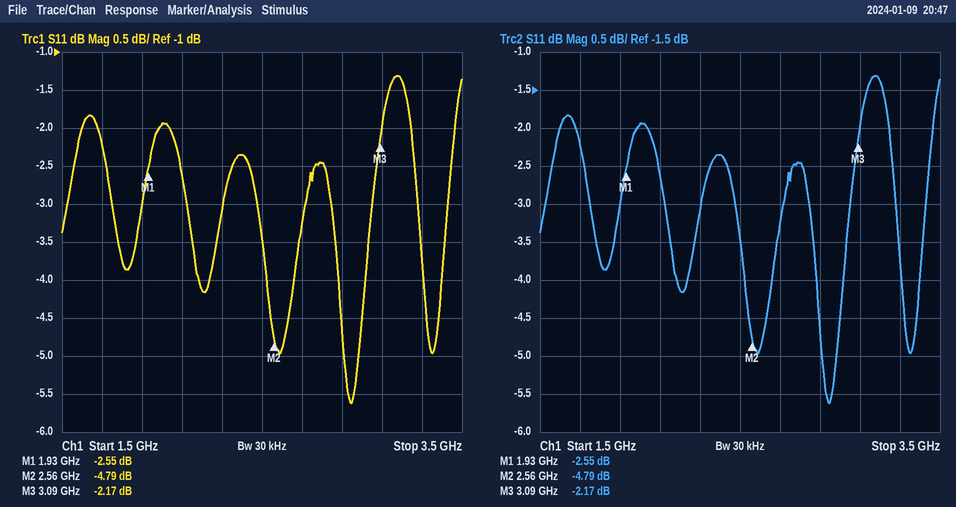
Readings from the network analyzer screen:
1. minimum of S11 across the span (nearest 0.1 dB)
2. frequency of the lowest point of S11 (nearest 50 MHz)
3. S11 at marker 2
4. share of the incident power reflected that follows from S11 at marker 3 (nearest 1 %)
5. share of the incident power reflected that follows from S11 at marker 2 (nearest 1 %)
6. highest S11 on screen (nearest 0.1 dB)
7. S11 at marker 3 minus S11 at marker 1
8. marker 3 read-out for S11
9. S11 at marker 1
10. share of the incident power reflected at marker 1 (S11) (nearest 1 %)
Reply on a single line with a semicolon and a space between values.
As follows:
-5.6 dB; 2.95 GHz; -4.79 dB; 61 %; 33 %; -1.3 dB; 0.38 dB; -2.17 dB; -2.55 dB; 56 %
